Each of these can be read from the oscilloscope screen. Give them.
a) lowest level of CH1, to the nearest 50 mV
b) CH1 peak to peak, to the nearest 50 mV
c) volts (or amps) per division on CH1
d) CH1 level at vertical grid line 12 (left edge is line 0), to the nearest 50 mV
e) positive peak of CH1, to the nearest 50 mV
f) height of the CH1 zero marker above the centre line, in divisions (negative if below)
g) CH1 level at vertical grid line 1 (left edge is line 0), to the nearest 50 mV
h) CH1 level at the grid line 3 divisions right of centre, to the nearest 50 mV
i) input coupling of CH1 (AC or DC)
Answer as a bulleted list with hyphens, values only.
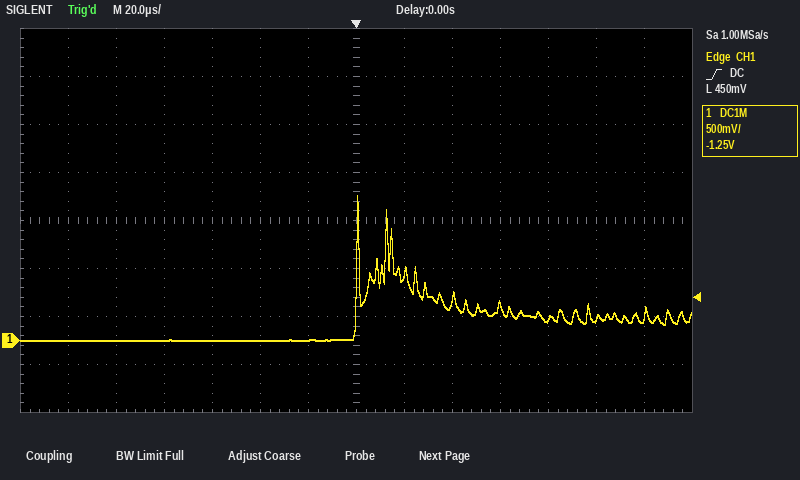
- 0 mV
- 1.50 V
- 500 mV
- 250 mV
- 1.50 V
- -2.5 div
- 0 mV
- 350 mV
- DC
